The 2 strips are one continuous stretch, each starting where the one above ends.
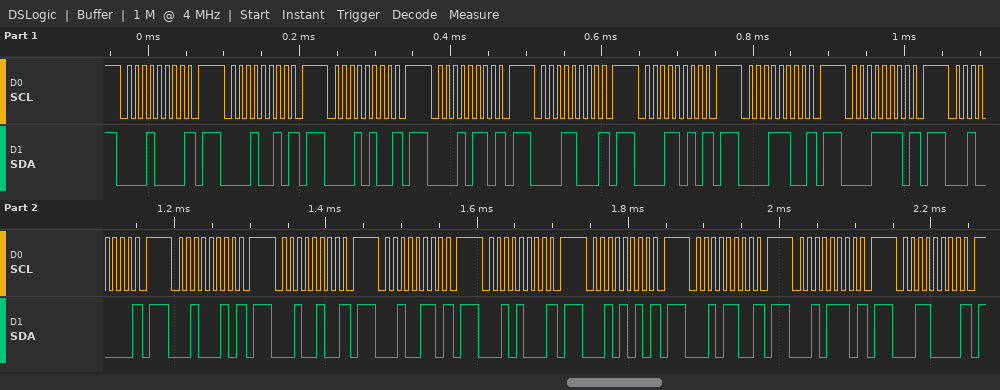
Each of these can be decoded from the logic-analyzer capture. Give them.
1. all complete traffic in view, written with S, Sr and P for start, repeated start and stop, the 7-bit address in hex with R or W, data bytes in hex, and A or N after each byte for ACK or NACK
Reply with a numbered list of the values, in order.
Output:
1. S 08W N P S 09W N P S 0AW N P S 0BW N P S 0CW N P S 0DW N P S 0EW N P S 0FW N P S 10W N P S 11W N P S 12W N P S 13W N P S 14W N P S 15W N P S 16W N P S 17W N P S 18W N P
